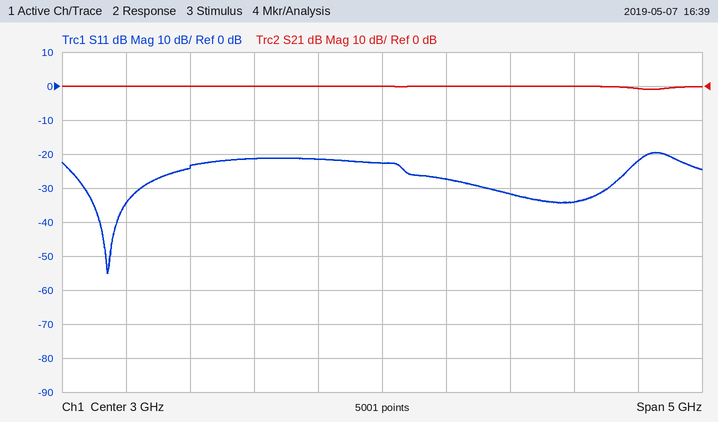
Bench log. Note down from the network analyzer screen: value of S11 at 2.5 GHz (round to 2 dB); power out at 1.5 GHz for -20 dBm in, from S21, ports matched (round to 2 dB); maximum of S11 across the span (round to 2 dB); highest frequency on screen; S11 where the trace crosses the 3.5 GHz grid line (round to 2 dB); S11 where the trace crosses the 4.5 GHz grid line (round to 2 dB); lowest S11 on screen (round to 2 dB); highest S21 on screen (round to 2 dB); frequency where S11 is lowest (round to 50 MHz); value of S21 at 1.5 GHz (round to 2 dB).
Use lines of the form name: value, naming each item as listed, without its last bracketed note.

value of S11 at 2.5 GHz: -22 dB
power out at 1.5 GHz for -20 dBm in, from S21, ports matched: -20 dBm
maximum of S11 across the span: -20 dB
highest frequency on screen: 5.5 GHz
S11 where the trace crosses the 3.5 GHz grid line: -28 dB
S11 where the trace crosses the 4.5 GHz grid line: -34 dB
lowest S11 on screen: -56 dB
highest S21 on screen: 0 dB
frequency where S11 is lowest: 850 MHz
value of S21 at 1.5 GHz: 0 dB
